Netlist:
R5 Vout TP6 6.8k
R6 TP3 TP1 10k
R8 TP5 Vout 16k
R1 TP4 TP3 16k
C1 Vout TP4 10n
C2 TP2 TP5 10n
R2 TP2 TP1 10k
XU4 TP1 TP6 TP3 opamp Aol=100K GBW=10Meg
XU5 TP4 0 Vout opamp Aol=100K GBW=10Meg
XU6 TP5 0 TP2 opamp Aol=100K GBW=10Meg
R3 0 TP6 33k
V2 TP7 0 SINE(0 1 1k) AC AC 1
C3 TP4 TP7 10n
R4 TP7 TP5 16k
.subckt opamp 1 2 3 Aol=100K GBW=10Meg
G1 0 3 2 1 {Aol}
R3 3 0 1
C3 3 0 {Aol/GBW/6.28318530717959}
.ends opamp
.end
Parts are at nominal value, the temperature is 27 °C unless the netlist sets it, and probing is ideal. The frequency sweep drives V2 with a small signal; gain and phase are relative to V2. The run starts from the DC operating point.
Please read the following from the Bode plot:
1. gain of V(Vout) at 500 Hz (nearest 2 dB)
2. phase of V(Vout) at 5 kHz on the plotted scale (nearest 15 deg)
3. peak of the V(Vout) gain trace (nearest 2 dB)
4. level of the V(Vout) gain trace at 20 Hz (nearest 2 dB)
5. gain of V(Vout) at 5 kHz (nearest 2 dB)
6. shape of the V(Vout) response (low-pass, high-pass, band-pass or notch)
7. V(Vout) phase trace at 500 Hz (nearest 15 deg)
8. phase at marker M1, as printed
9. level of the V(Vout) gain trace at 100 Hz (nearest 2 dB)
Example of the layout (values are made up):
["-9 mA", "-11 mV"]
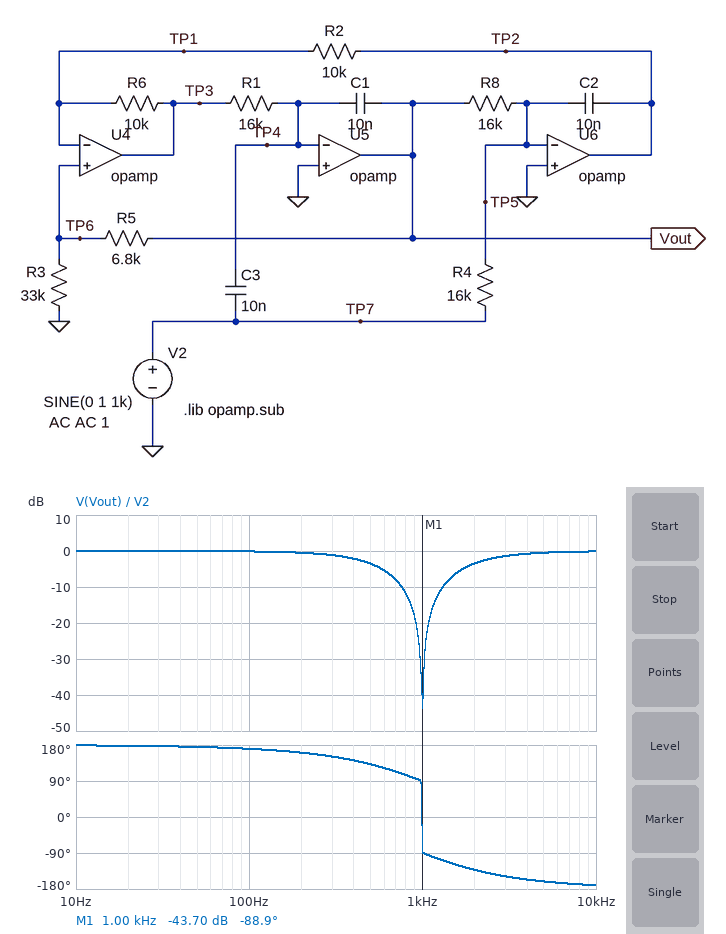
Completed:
["-4 dB", "-165 deg", "0 dB", "0 dB", "0 dB", "notch", "135 deg", "-88.9 deg", "0 dB"]
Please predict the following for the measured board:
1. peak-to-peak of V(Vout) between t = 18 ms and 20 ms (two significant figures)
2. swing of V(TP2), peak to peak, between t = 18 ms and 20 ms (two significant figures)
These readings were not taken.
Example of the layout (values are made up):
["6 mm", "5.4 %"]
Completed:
["13 mV", "2.0 V"]
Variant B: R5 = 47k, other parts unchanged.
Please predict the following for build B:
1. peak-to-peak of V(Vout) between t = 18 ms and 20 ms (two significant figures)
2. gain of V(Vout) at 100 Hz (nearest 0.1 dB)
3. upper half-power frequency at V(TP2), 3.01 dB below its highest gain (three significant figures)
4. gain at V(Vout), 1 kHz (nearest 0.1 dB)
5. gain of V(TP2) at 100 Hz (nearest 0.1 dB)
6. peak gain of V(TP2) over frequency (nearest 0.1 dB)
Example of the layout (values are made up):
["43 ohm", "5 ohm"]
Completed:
["26 mV", "0 dB", "1.18 kHz", "-37.6 dB", "-1.6 dB", "0.8 dB"]
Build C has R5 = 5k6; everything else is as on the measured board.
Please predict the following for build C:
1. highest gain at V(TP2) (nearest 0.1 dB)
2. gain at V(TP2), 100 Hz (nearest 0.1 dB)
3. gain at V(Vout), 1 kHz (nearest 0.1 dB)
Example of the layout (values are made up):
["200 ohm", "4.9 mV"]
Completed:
["4.7 dB", "4.6 dB", "-44.0 dB"]
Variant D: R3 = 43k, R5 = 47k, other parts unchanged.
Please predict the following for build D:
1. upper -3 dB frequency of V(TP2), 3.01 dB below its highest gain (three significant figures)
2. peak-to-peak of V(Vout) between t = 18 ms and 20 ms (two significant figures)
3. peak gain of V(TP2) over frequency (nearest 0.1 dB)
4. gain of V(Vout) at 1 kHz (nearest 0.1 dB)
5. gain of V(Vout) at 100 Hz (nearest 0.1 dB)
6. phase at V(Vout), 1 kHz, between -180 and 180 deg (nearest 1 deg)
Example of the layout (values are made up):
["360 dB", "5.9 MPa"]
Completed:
["1.17 kHz", "23 mV", "1.1 dB", "-38.9 dB", "0 dB", "-89 deg"]
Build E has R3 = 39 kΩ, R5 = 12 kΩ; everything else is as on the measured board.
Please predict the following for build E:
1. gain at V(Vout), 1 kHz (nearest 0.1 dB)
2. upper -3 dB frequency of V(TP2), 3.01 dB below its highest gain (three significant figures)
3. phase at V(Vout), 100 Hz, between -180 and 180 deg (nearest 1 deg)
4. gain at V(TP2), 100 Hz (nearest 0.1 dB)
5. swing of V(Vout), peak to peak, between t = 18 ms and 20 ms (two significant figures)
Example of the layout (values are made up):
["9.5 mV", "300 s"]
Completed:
["-43.0 dB", "914 Hz", "171 deg", "3.7 dB", "14 mV"]
